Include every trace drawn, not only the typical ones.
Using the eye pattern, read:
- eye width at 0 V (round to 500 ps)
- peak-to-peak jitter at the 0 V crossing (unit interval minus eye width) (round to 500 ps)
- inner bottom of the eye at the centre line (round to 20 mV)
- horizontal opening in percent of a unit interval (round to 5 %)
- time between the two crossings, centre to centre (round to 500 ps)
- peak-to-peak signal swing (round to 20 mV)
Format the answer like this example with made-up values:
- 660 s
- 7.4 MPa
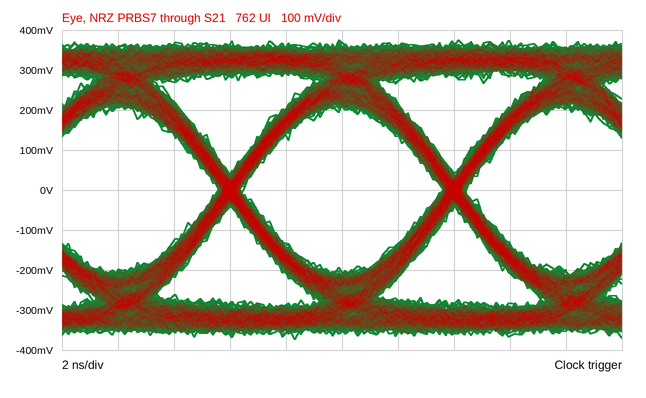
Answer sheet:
- 7.0 ns
- 1.0 ns
- -200 mV
- 90 %
- 8.0 ns
- 740 mV
